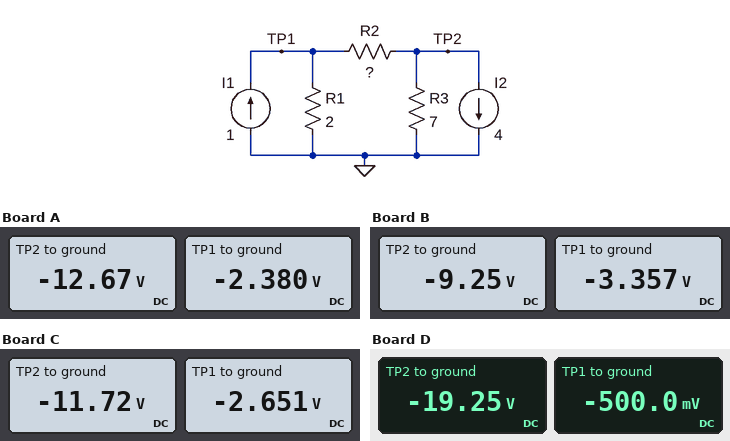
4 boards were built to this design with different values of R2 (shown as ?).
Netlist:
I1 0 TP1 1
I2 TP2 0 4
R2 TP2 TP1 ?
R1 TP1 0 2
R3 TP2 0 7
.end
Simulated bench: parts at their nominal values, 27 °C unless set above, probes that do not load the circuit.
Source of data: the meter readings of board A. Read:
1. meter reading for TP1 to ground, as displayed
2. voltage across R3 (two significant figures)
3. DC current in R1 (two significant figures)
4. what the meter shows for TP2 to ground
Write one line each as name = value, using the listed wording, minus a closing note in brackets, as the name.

meter reading for TP1 to ground, as displayed = -2.380 V
voltage across R3 = 13 V
DC current in R1 = 1.2 A
what the meter shows for TP2 to ground = -12.67 V
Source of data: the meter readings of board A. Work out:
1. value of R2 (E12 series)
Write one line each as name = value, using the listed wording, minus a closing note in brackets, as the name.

value of R2 = 4.7 Ω
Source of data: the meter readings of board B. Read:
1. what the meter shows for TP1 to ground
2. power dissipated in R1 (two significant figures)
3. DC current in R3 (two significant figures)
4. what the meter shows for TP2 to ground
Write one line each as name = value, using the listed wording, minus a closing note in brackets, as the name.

what the meter shows for TP1 to ground = -3.357 V
power dissipated in R1 = 5.6 W
DC current in R3 = 1.3 A
what the meter shows for TP2 to ground = -9.25 V
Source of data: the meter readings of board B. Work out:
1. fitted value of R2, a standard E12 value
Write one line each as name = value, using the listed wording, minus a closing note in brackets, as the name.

fitted value of R2, a standard E12 value = 2.2 Ω
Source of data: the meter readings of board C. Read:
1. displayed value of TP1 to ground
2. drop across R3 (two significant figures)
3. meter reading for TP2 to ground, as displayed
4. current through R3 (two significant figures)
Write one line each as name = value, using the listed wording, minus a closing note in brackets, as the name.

displayed value of TP1 to ground = -2.651 V
drop across R3 = 12 V
meter reading for TP2 to ground, as displayed = -11.72 V
current through R3 = 1.7 A
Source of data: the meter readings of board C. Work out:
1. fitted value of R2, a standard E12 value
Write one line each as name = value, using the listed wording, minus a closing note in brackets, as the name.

fitted value of R2, a standard E12 value = 3.9 Ω
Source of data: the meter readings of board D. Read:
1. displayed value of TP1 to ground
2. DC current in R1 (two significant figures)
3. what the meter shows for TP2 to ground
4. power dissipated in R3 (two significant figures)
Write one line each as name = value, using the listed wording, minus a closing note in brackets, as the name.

displayed value of TP1 to ground = -500.0 mV
DC current in R1 = 250 mA
what the meter shows for TP2 to ground = -19.25 V
power dissipated in R3 = 53 W
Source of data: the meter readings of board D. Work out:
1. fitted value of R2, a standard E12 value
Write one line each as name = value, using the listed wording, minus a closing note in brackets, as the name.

fitted value of R2, a standard E12 value = 15 Ω
